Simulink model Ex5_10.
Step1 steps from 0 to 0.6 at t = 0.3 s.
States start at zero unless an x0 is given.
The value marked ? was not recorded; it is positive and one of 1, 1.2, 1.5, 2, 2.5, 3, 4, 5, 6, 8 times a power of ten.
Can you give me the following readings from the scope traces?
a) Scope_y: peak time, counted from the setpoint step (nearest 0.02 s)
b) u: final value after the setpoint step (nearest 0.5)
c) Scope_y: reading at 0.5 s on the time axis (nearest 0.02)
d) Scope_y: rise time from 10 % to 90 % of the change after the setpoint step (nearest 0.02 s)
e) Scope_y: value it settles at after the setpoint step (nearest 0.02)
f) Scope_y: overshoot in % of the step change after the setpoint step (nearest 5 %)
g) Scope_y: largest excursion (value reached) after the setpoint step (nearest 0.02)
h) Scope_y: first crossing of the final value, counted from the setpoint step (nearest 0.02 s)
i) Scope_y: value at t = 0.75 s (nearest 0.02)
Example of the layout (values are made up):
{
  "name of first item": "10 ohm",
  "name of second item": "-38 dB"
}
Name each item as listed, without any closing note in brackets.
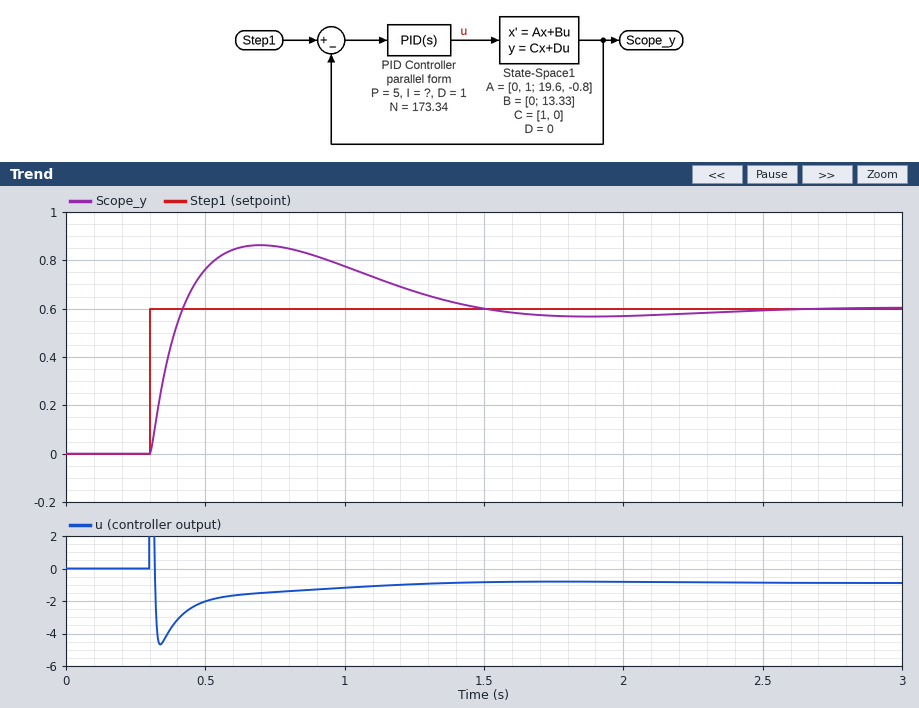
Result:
{
  "Scope_y: peak time, counted from the setpoint step": "0.40 s",
  "u: final value after the setpoint step": "-1.0",
  "Scope_y: reading at 0.5 s on the time axis": "0.76",
  "Scope_y: rise time from 10 % to 90 % of the change after the setpoint step": "0.08 s",
  "Scope_y: value it settles at after the setpoint step": "0.60",
  "Scope_y: overshoot in % of the step change after the setpoint step": "45 %",
  "Scope_y: largest excursion (value reached) after the setpoint step": "0.86",
  "Scope_y: first crossing of the final value, counted from the setpoint step": "0.12 s",
  "Scope_y: value at t = 0.75 s": "0.86"
}
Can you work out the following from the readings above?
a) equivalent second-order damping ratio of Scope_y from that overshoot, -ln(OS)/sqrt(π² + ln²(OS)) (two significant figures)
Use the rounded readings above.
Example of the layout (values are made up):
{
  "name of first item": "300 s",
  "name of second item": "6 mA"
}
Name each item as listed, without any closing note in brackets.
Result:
{
  "equivalent second-order damping ratio of Scope_y from that overshoot, -ln(OS)/sqrt(π² + ln²(OS))": "0.25"
}
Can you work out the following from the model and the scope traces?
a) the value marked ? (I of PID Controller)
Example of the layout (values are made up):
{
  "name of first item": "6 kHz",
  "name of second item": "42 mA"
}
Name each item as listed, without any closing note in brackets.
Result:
{
  "the value marked ?": "8"
}
